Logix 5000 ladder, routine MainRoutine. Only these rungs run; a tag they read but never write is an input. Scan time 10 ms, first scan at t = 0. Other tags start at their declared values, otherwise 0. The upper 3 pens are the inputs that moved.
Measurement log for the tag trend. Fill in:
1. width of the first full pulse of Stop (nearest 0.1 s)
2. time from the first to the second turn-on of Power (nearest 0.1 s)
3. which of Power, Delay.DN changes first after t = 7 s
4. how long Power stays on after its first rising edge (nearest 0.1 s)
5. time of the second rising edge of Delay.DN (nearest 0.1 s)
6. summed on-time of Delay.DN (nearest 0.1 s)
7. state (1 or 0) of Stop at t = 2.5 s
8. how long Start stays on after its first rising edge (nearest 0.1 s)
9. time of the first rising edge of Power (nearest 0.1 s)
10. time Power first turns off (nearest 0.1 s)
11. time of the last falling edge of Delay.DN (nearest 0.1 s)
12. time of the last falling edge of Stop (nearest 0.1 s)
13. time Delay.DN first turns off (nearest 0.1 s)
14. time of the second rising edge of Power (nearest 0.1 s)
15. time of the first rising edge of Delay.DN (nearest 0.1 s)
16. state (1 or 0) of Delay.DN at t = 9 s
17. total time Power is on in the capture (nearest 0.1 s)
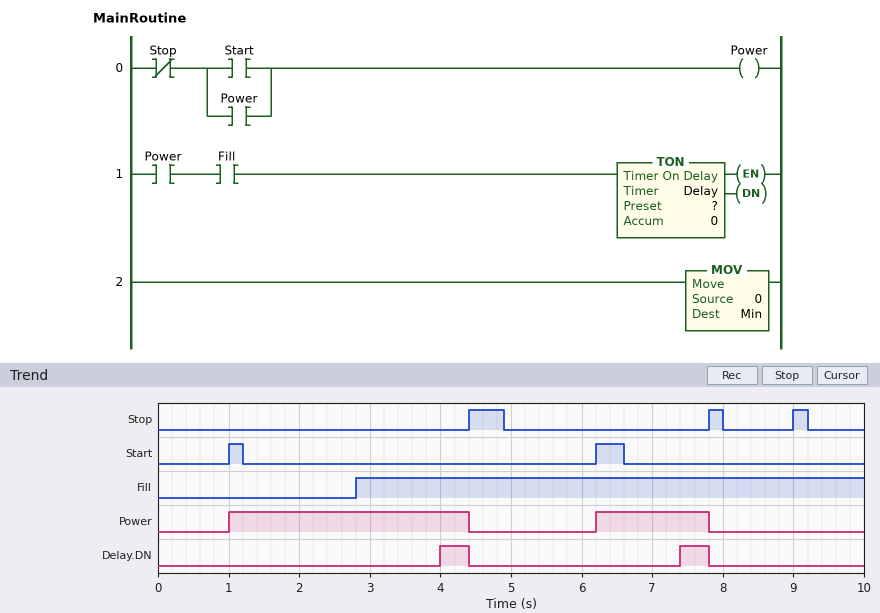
0.5 s
5.2 s
Delay.DN
3.4 s
7.4 s
0.8 s
0
0.2 s
1.0 s
4.4 s
7.8 s
9.2 s
4.4 s
6.2 s
4.0 s
0
5.0 s
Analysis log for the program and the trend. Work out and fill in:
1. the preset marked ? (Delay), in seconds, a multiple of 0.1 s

1.2 s
